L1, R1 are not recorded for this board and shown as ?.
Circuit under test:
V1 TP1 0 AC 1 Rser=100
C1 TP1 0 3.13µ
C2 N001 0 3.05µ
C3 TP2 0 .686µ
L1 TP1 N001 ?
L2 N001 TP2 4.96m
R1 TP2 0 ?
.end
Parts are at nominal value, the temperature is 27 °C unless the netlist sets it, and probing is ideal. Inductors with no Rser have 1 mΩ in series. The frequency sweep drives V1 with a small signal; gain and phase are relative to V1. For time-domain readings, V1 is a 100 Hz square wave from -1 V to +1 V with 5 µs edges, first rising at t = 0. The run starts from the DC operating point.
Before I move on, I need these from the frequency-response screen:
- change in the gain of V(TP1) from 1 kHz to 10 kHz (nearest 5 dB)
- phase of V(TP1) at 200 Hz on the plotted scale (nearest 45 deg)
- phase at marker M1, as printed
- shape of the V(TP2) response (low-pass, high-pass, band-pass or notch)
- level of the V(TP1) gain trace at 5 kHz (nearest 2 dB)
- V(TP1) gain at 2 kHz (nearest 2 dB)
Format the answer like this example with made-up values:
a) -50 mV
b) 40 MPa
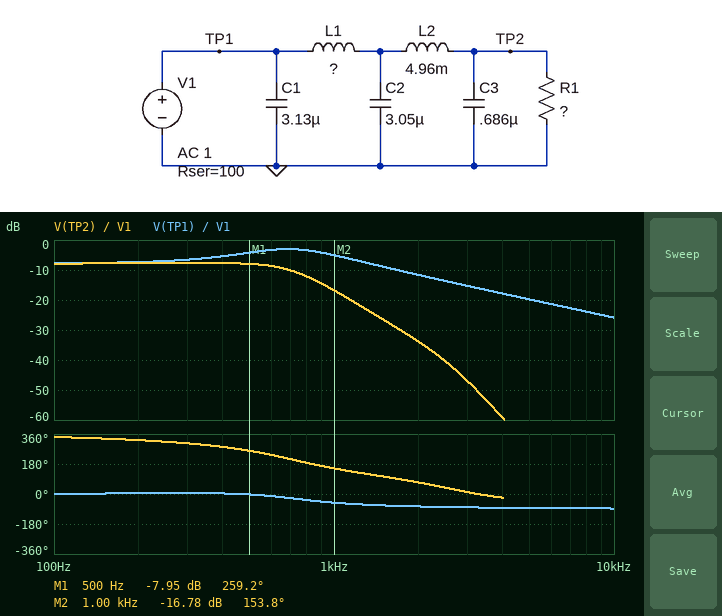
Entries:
a) -20 dB
b) 0 deg
c) 259.2 deg
d) low-pass
e) -20 dB
f) -12 dB
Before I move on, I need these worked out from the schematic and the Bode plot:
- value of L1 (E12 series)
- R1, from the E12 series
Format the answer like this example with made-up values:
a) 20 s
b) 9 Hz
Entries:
a) 33 mH
b) 68 Ω
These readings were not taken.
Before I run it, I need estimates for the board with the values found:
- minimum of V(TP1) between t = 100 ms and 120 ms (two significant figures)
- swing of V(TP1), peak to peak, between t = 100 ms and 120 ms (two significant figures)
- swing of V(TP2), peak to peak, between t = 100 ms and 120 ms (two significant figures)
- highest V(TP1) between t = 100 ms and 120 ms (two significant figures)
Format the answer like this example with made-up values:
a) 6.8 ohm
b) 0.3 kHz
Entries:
a) -730 mV
b) 1.5 V
c) 970 mV
d) 730 mV
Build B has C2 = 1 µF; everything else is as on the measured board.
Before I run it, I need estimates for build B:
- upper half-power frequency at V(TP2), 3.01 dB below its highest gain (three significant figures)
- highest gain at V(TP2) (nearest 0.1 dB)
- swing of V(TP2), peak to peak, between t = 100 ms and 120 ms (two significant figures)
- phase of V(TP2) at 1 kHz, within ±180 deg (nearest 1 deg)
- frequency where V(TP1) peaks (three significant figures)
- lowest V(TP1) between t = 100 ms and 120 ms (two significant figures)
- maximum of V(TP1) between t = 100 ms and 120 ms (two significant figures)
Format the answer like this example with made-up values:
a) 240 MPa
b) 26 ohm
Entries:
a) 710 Hz
b) -7.7 dB
c) 930 mV
d) -164 deg
e) 603 Hz
f) -760 mV
g) 760 mV
